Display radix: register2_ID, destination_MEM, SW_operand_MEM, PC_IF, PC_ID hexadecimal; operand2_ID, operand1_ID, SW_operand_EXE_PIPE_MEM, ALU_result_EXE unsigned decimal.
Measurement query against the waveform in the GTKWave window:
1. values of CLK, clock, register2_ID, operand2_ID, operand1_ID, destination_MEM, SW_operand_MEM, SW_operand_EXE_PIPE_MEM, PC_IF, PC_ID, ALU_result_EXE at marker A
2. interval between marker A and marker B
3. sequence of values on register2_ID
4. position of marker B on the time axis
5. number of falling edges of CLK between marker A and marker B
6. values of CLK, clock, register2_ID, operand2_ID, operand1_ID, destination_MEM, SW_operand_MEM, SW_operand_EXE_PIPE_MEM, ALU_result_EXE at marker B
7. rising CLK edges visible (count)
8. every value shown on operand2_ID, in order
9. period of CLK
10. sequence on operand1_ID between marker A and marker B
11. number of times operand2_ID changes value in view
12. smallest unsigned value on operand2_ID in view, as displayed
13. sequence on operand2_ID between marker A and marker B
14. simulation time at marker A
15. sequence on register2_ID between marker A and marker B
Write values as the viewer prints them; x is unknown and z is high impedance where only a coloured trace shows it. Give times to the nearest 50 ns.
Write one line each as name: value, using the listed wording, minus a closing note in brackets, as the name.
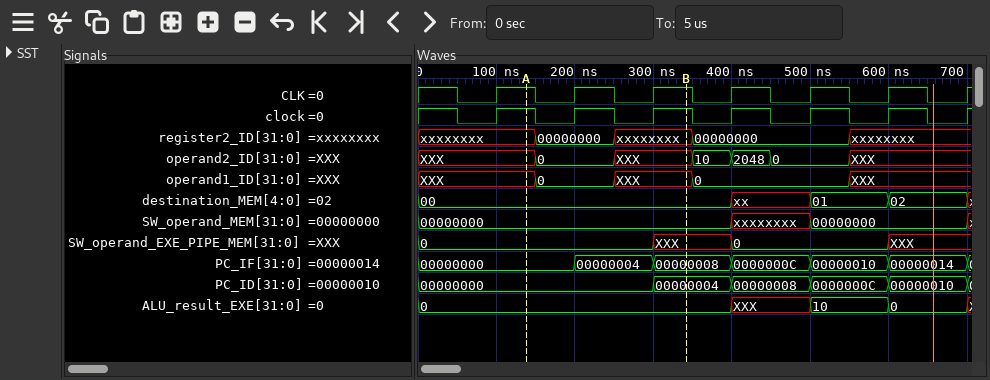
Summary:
values of CLK, clock, register2_ID, operand2_ID, operand1_ID, destination_MEM, SW_operand_MEM, SW_operand_EXE_PIPE_MEM, PC_IF, PC_ID, ALU_result_EXE at marker A: CLK=1, clock=1, register2_ID=xxxxxxxx, operand2_ID=XXX, operand1_ID=XXX, destination_MEM=00, SW_operand_MEM=00000000, SW_operand_EXE_PIPE_MEM=0, PC_IF=00000000, PC_ID=00000000, ALU_result_EXE=0
interval between marker A and marker B: 200 ns
sequence of values on register2_ID: xxxxxxxx, 00000000, xxxxxxxx, 00000000, xxxxxxxx
position of marker B on the time axis: 350 ns
number of falling edges of CLK between marker A and marker B: 2
values of CLK, clock, register2_ID, operand2_ID, operand1_ID, destination_MEM, SW_operand_MEM, SW_operand_EXE_PIPE_MEM, ALU_result_EXE at marker B: CLK=1, clock=1, register2_ID=xxxxxxxx, operand2_ID=XXX, operand1_ID=XXX, destination_MEM=00, SW_operand_MEM=00000000, SW_operand_EXE_PIPE_MEM=XXX, ALU_result_EXE=0
rising CLK edges visible: 7
every value shown on operand2_ID, in order: XXX, 0, XXX, 10, 2048, 0, XXX
period of CLK: 100 ns
sequence on operand1_ID between marker A and marker B: XXX, 0, XXX
number of times operand2_ID changes value in view: 6
smallest unsigned value on operand2_ID in view, as displayed: 0
sequence on operand2_ID between marker A and marker B: XXX, 0, XXX
simulation time at marker A: 150 ns
sequence on register2_ID between marker A and marker B: xxxxxxxx, 00000000, xxxxxxxx
